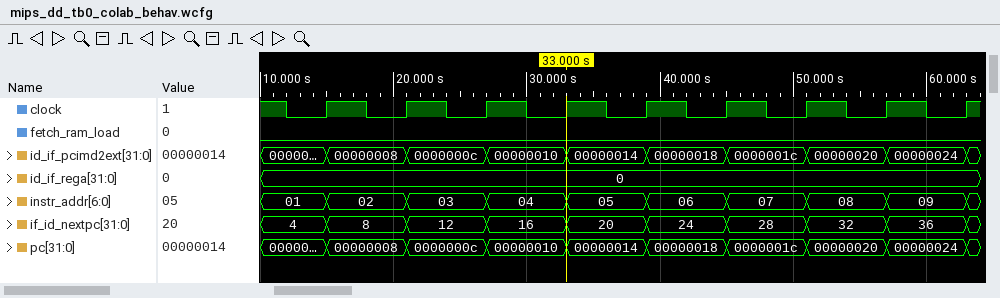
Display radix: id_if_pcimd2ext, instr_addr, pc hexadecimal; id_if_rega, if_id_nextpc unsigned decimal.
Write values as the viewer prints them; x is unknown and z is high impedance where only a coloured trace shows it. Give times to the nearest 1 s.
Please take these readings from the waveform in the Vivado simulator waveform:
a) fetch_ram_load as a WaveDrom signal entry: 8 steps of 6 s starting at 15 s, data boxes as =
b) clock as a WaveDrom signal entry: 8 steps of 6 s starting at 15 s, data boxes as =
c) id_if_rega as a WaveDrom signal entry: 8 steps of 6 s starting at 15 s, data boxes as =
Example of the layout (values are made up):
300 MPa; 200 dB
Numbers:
{name: 'fetch_ram_load', wave: '0.......'}; {name: 'clock', wave: 'p.......'}; {name: 'id_if_rega', wave: '=.......', data: '0'}
